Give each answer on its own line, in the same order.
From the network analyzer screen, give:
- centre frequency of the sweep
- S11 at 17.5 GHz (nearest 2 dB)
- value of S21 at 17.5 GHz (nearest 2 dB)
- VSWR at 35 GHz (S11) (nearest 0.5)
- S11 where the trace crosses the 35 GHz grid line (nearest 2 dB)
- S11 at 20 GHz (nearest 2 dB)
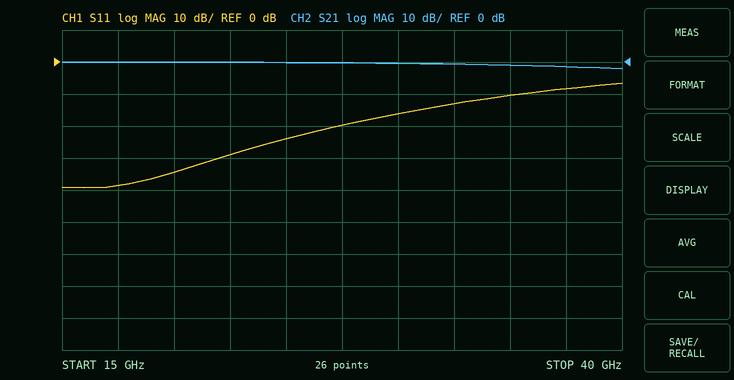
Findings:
27.5 GHz
-38 dB
0 dB
2.0
-10 dB
-34 dB
